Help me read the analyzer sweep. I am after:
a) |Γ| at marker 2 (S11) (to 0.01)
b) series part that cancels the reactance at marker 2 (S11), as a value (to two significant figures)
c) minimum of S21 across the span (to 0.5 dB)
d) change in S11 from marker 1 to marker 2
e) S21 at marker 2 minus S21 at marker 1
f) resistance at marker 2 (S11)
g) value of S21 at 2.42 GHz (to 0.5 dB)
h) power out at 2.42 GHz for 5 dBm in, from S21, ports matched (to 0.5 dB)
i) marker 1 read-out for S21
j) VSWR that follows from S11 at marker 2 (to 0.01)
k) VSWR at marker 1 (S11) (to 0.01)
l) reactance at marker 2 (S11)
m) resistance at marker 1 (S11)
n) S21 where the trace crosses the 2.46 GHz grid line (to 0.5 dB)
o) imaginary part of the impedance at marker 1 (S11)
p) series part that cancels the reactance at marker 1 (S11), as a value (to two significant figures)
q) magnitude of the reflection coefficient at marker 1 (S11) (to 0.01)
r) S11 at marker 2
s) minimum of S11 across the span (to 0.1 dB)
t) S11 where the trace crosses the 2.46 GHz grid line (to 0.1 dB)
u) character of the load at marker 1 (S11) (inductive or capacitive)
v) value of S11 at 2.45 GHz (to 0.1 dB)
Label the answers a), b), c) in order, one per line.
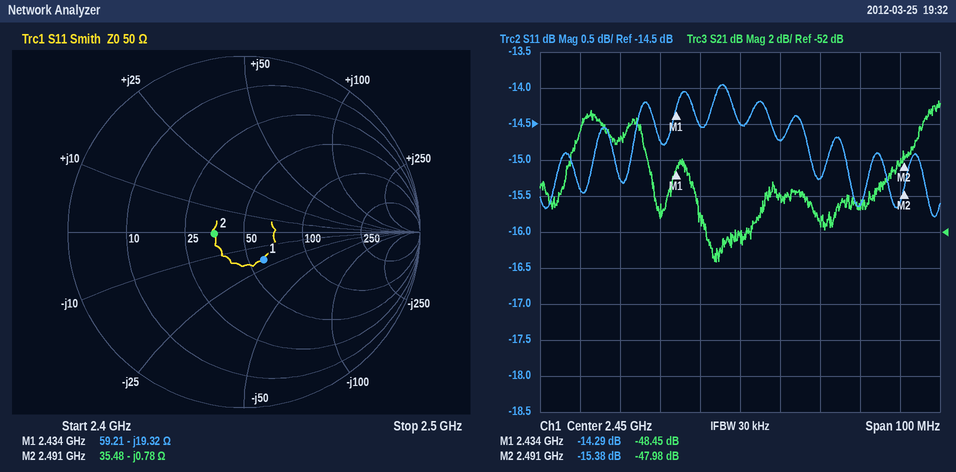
a) 0.17
b) 50 pH
c) -53.5 dB
d) -1.09 dB
e) 0.47 dB
f) 35.48 Ω
g) -47.0 dB
h) -42.0 dBm
i) -48.45 dB
j) 1.41
k) 1.48
l) -0.78 Ω
m) 59.21 Ω
n) -50.0 dB
o) -19.32 Ω
p) 1.3 nH
q) 0.19
r) -15.38 dB
s) -15.8 dB
t) -14.7 dB
u) capacitive
v) -14.5 dB
